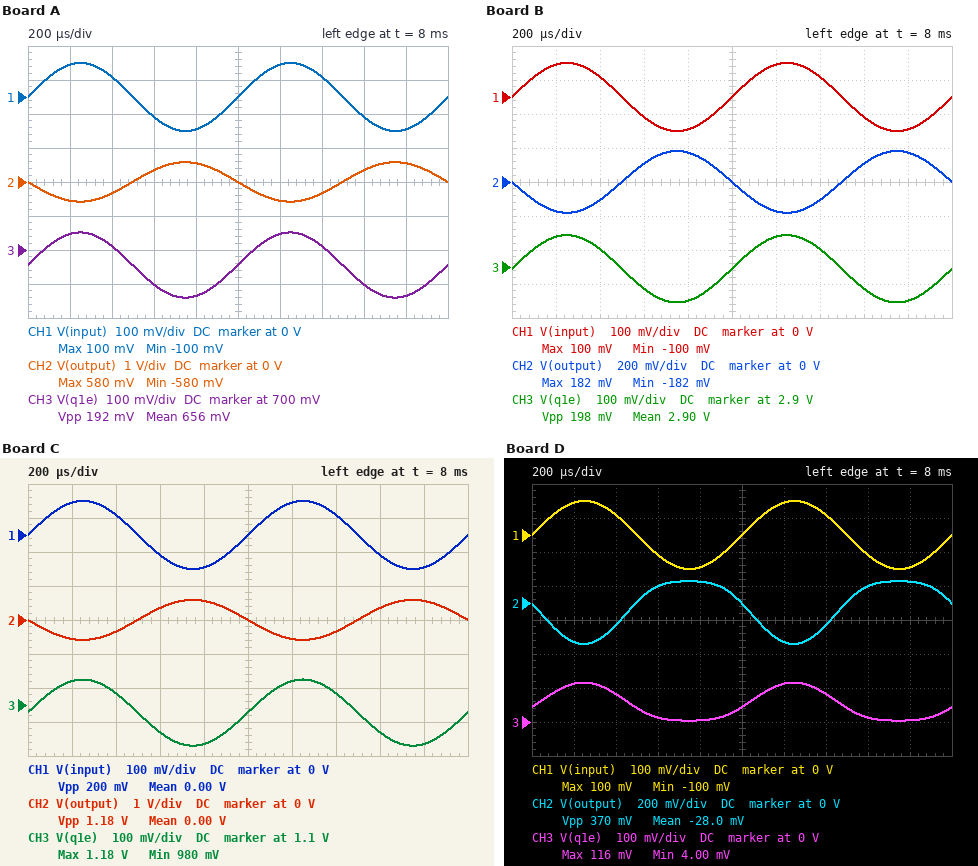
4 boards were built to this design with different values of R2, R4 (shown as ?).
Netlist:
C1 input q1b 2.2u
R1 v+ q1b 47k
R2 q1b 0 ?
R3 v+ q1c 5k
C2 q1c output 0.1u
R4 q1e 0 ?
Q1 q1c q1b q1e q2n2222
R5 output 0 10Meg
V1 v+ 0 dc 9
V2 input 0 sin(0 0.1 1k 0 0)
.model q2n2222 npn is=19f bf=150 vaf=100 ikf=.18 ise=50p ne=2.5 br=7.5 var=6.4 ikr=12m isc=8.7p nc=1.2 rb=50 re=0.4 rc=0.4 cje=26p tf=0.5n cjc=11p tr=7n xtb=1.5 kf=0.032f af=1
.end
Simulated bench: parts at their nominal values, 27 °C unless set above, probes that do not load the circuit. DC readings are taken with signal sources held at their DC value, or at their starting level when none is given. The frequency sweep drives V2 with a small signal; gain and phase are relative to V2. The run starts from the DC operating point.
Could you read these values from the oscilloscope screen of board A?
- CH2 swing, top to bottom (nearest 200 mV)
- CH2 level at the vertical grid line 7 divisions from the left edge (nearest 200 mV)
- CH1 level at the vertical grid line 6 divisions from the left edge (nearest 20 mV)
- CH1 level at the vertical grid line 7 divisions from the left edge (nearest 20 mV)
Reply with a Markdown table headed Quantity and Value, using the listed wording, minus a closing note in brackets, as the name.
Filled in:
| Quantity | Value |
|---|---|
| CH2 swing, top to bottom | 1.2 V |
| CH2 level at the vertical grid line 7 divisions from the left edge | -400 mV |
| CH1 level at the vertical grid line 6 divisions from the left edge | 100 mV |
| CH1 level at the vertical grid line 7 divisions from the left edge | 60 mV |
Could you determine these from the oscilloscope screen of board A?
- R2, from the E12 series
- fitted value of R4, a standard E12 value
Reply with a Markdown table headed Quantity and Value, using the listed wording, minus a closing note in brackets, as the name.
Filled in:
| Quantity | Value |
|---|---|
| R2, from the E12 series | 8.2 kΩ |
| fitted value of R4, a standard E12 value | 820 Ω |
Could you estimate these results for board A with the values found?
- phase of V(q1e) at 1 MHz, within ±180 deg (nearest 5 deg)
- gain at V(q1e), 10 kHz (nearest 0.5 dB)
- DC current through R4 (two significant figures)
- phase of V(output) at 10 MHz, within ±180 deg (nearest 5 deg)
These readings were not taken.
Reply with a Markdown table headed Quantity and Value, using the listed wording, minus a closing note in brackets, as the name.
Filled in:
| Quantity | Value |
|---|---|
| phase of V(q1e) at 1 MHz, within ±180 deg | 0 deg |
| gain at V(q1e), 10 kHz | -0.5 dB |
| DC current through R4 | 800 µA |
| phase of V(output) at 10 MHz, within ±180 deg | 90 deg |
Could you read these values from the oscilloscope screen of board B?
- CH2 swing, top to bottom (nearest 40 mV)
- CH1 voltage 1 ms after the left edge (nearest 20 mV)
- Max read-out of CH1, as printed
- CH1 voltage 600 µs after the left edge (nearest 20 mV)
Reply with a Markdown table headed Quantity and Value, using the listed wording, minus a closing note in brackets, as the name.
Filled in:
| Quantity | Value |
|---|---|
| CH2 swing, top to bottom | 360 mV |
| CH1 voltage 1 ms after the left edge | 0 V |
| Max read-out of CH1, as printed | 100 mV |
| CH1 voltage 600 µs after the left edge | -60 mV |
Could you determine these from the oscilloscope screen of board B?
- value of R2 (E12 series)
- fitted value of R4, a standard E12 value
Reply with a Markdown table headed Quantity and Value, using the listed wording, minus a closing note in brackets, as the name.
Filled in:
| Quantity | Value |
|---|---|
| value of R2 | 33 kΩ |
| fitted value of R4, a standard E12 value | 2.7 kΩ |
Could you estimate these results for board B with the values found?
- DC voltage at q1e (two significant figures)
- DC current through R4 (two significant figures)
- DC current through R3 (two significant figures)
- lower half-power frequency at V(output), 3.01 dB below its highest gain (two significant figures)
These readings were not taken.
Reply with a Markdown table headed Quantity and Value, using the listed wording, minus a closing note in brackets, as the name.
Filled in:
| Quantity | Value |
|---|---|
| DC voltage at q1e | 2.9 V |
| DC current through R4 | 1.1 mA |
| DC current through R3 | 1.1 mA |
| lower half-power frequency at V(output), 3.01 dB below its highest gain | 4.0 Hz |
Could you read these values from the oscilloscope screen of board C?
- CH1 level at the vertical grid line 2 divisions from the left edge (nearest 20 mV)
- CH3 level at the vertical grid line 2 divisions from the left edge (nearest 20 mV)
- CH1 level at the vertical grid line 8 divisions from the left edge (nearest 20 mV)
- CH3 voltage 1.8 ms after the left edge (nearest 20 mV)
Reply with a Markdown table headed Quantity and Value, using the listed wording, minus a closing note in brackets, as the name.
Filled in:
| Quantity | Value |
|---|---|
| CH1 level at the vertical grid line 2 divisions from the left edge | 60 mV |
| CH3 level at the vertical grid line 2 divisions from the left edge | 1.14 V |
| CH1 level at the vertical grid line 8 divisions from the left edge | -60 mV |
| CH3 voltage 1.8 ms after the left edge | 980 mV |
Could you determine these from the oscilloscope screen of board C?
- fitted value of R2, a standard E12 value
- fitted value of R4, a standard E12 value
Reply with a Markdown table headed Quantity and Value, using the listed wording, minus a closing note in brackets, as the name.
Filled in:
| Quantity | Value |
|---|---|
| fitted value of R2, a standard E12 value | 12 kΩ |
| fitted value of R4, a standard E12 value | 820 Ω |
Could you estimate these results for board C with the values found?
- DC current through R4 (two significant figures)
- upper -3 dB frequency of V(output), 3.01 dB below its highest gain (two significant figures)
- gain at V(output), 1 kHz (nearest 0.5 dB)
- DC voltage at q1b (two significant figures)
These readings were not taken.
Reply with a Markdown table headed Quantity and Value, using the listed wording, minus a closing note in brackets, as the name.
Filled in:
| Quantity | Value |
|---|---|
| DC current through R4 | 1.3 mA |
| upper -3 dB frequency of V(output), 3.01 dB below its highest gain | 3.5 MHz |
| gain at V(output), 1 kHz | 15.5 dB |
| DC voltage at q1b | 1.7 V |
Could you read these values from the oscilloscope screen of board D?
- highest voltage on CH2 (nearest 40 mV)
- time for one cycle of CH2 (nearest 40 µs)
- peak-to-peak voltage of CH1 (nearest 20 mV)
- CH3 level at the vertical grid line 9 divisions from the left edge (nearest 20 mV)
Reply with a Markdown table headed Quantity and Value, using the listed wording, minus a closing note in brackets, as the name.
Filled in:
| Quantity | Value |
|---|---|
| highest voltage on CH2 | 120 mV |
| time for one cycle of CH2 | 1.00 ms |
| peak-to-peak voltage of CH1 | 200 mV |
| CH3 level at the vertical grid line 9 divisions from the left edge | 0 V |
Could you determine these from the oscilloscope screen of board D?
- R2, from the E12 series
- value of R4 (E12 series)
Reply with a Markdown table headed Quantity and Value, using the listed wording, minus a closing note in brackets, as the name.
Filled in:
| Quantity | Value |
|---|---|
| R2, from the E12 series | 3.3 kΩ |
| value of R4 | 1.5 kΩ |
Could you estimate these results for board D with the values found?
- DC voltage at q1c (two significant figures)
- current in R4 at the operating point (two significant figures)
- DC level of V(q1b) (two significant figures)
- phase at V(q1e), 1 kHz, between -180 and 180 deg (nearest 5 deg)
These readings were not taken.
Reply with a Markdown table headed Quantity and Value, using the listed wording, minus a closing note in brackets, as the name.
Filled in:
| Quantity | Value |
|---|---|
| DC voltage at q1c | 8.9 V |
| current in R4 at the operating point | 29 µA |
| DC level of V(q1b) | 590 mV |
| phase at V(q1e), 1 kHz, between -180 and 180 deg | 0 deg |
